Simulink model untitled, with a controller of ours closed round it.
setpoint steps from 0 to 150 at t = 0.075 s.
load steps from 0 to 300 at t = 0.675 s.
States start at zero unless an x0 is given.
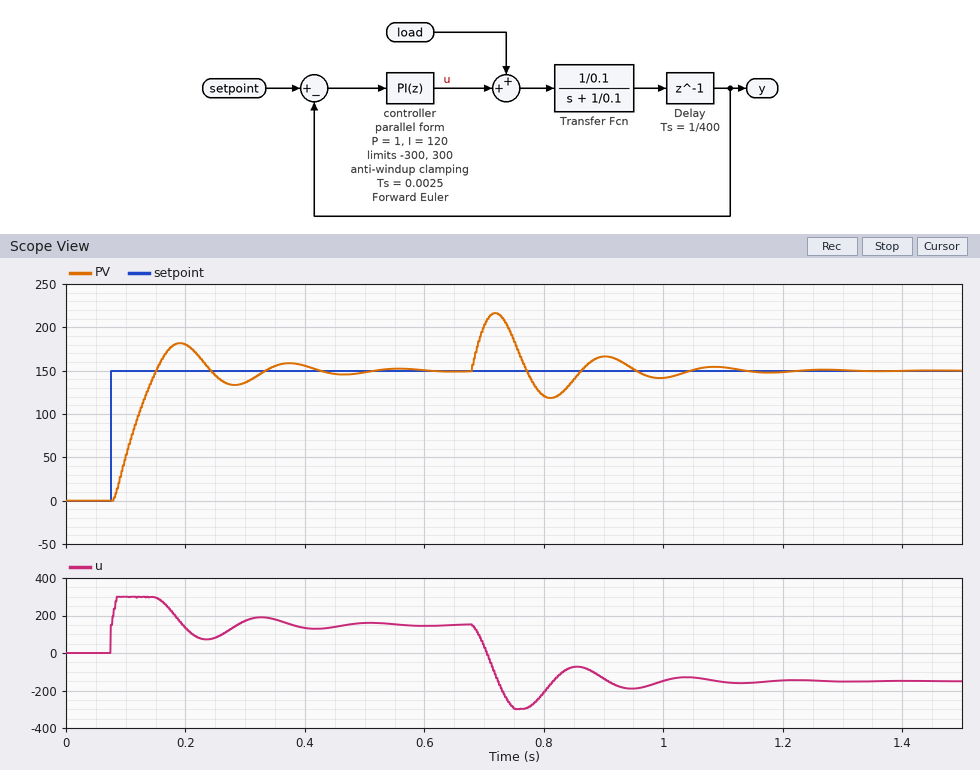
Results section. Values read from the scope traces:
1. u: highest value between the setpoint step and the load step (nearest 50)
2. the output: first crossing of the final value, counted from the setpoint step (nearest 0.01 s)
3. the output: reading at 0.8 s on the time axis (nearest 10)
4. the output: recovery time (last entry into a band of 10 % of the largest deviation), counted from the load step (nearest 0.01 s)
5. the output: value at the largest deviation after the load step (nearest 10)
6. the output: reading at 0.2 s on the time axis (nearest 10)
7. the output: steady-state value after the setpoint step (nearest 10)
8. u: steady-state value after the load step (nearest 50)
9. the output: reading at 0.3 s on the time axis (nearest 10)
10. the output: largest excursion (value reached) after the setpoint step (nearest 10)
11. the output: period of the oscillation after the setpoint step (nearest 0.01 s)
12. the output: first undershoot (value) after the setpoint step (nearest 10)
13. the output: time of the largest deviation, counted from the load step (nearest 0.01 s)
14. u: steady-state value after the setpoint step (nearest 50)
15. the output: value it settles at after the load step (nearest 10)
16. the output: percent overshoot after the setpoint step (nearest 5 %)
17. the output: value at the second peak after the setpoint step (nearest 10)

300
0.08 s
120
0.34 s
220
180
150
-150
140
180
0.18 s
130
0.04 s
150
150
20 %
160
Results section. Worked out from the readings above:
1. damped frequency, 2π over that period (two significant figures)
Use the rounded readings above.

35 rad/s
